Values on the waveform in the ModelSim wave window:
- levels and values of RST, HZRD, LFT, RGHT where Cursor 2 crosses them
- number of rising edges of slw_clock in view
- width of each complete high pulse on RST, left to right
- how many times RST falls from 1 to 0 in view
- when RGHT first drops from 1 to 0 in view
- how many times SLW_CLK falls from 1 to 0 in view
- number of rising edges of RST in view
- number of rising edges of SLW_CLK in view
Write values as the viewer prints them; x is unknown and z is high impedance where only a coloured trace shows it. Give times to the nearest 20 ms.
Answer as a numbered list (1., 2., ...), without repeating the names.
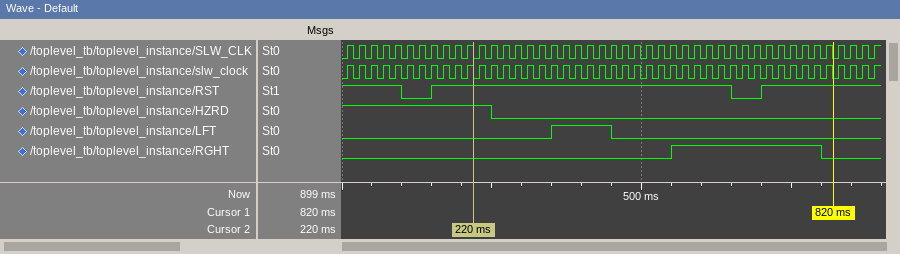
1. RST=1, HZRD=1, LFT=0, RGHT=0
2. 45
3. 500 ms
4. 2
5. 800 ms
6. 44
7. 2
8. 45
